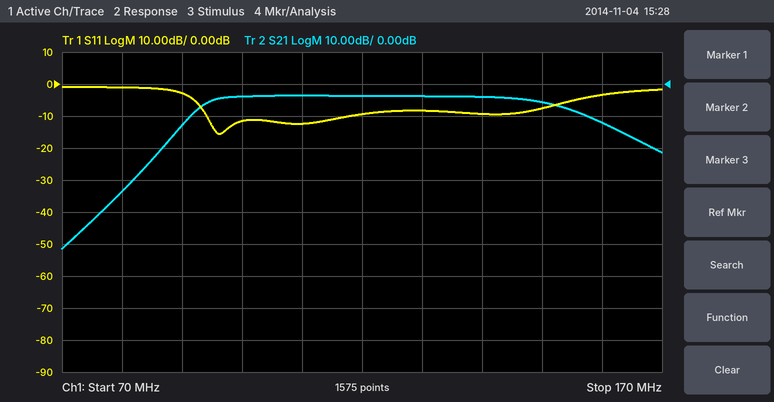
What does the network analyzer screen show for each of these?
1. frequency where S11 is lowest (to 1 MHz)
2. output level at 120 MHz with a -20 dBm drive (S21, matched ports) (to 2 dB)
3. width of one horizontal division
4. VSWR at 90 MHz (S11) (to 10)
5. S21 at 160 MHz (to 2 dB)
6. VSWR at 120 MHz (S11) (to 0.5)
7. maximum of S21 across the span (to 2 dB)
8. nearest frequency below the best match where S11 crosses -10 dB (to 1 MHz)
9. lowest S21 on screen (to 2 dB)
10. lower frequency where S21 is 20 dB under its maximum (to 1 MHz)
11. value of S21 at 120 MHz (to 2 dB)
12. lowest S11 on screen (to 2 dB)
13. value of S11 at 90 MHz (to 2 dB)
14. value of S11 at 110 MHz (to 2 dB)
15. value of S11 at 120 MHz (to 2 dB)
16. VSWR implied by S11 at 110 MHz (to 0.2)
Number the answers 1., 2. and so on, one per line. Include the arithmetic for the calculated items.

1. 96 MHz
2. -20 dBm + (-4 dB) = -24 dBm
3. 10 MHz
4. |Γ| = 10^(-2/20) = 0.7943; VSWR = (1 + 0.7943)/(1 − 0.7943) ≈ 8.72, so 10 to the nearest 10
5. -12 dB
6. |Γ| = 10^(-10/20) = 0.3162; VSWR = (1 + 0.3162)/(1 − 0.3162) ≈ 1.92, so 2.0 to the nearest 0.5
7. -4 dB
8. 94 MHz
9. -52 dB
10. 85 MHz
11. -4 dB
12. -16 dB
13. -2 dB
14. -12 dB
15. -10 dB
16. |Γ| = 10^(-12/20) = 0.2512; VSWR = (1 + 0.2512)/(1 − 0.2512) ≈ 1.67, so 1.6 to the nearest 0.2
